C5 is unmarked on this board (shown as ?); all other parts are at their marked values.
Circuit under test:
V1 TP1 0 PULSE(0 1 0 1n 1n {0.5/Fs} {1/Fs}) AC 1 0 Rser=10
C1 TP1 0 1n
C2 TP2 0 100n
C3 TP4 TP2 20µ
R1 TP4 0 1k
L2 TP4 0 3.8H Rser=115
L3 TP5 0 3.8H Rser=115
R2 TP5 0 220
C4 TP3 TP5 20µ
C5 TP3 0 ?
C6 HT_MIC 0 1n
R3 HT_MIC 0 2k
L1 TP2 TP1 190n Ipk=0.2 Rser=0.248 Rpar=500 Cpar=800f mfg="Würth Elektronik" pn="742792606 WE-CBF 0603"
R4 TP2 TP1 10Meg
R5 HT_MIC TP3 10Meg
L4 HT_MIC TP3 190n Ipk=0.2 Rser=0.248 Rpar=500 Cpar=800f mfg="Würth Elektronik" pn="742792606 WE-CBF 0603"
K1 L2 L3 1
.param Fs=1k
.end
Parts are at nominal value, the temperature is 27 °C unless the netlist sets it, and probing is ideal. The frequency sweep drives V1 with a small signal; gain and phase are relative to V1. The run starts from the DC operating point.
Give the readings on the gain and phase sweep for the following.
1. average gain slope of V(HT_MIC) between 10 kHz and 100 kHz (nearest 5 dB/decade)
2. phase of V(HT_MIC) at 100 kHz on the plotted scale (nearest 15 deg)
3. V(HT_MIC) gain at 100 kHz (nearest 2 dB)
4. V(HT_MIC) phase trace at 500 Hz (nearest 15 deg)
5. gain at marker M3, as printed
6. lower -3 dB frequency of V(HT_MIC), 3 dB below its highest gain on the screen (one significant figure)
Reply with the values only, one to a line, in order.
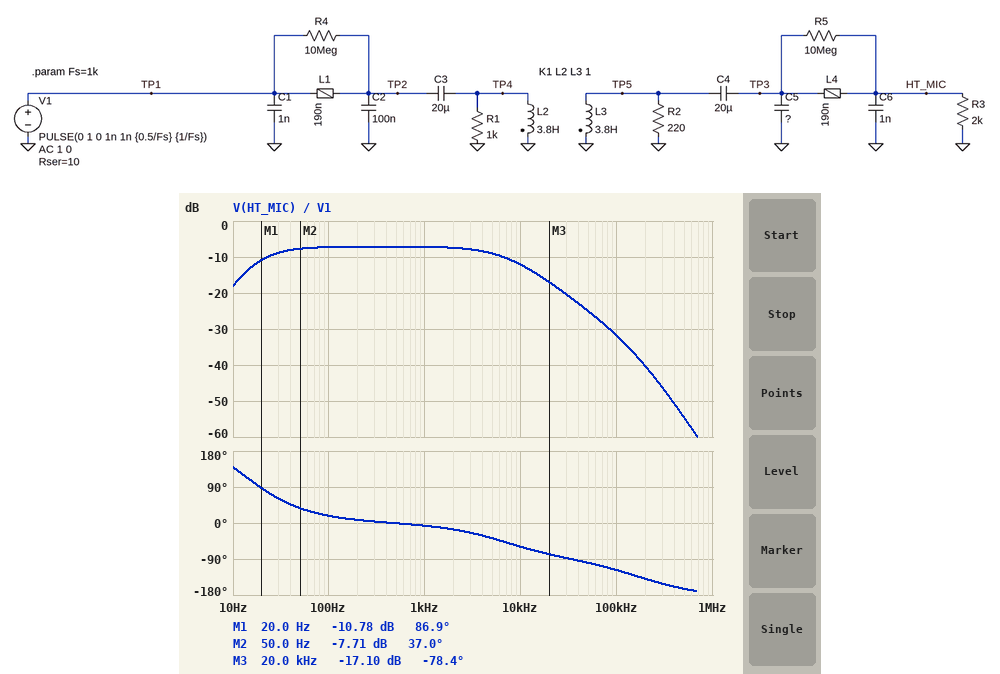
-20 dB/decade
-120 deg
-32 dB
0 deg
-17.10 dB
20 Hz
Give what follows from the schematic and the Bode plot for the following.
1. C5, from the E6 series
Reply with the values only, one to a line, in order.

220 nF
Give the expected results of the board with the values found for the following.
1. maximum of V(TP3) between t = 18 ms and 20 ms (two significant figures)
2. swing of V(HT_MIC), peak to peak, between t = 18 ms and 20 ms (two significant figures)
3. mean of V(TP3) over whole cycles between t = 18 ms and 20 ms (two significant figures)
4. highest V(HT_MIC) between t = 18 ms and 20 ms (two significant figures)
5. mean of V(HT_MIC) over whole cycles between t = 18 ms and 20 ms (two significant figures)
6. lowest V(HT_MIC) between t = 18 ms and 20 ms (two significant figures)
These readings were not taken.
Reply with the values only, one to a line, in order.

180 mV
450 mV
-43 mV
180 mV
-43 mV
-270 mV
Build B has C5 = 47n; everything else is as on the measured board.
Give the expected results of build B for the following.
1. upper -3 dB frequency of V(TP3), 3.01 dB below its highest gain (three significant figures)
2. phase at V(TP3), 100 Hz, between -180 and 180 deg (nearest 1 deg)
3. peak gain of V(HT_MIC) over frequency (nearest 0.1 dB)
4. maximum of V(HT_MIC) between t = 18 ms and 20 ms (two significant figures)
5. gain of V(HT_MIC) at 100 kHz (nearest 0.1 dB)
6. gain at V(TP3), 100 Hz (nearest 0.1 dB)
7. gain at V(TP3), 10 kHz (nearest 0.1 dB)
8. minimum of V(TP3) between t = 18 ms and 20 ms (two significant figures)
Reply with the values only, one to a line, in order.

29.6 kHz
19 deg
-7.0 dB
190 mV
-19.1 dB
-7.2 dB
-7.5 dB
-280 mV
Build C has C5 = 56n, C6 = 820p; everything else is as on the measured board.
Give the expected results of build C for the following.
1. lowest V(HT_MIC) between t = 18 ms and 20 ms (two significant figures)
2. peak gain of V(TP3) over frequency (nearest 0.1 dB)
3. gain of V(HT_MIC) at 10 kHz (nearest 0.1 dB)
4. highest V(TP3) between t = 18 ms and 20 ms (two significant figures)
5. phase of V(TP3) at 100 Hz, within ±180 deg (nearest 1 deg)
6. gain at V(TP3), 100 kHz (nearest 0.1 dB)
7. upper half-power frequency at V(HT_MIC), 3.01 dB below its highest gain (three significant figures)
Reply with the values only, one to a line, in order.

-280 mV
-7.0 dB
-7.6 dB
190 mV
19 deg
-20.4 dB
25.2 kHz
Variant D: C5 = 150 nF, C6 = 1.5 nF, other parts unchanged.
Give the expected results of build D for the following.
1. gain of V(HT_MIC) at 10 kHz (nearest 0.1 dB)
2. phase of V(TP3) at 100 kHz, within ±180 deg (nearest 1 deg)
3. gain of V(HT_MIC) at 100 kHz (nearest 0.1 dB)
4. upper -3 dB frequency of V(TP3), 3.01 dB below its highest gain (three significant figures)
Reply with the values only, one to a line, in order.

-10.2 dB
-116 deg
-28.7 dB
9.75 kHz
